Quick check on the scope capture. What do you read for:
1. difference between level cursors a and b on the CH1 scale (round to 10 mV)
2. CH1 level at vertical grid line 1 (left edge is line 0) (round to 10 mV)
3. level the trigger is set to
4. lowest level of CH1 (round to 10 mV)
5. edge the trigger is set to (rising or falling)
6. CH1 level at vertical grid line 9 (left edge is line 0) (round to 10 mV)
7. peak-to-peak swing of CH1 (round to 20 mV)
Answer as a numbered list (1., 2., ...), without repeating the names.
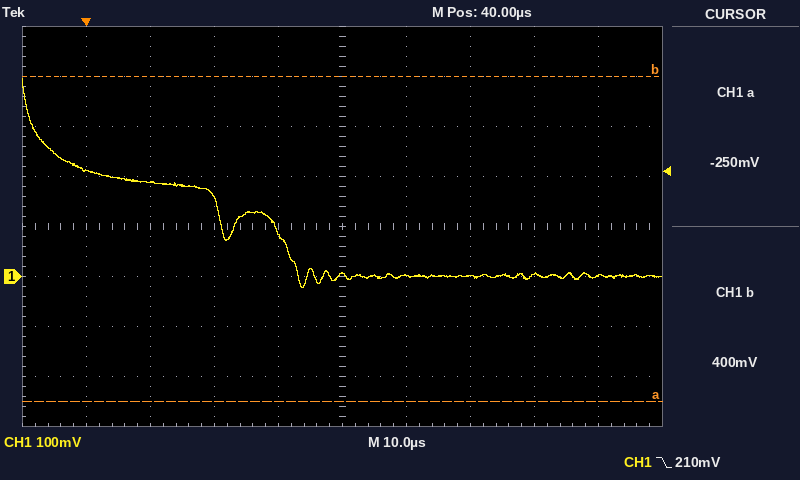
1. 650 mV
2. 210 mV
3. 210 mV
4. -20 mV
5. falling
6. 0 mV
7. 420 mV
